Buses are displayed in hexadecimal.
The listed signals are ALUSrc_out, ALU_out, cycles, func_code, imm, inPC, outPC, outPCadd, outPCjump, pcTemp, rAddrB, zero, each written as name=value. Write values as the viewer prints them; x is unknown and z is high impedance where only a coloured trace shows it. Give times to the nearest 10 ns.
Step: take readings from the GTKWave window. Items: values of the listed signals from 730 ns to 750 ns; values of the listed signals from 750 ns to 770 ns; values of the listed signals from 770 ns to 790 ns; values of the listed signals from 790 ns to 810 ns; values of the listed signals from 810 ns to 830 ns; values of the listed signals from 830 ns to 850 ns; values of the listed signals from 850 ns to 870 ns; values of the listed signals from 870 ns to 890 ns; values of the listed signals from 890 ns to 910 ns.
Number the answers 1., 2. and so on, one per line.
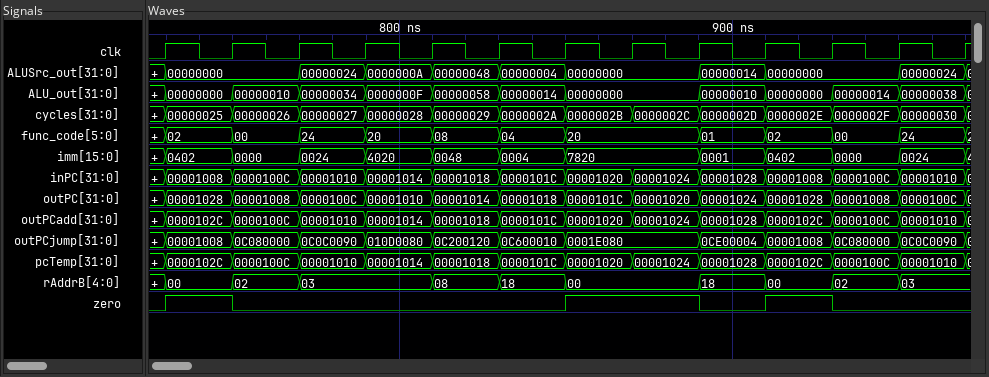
1. ALUSrc_out=00000000, ALU_out=00000000, cycles=00000025, func_code=02, imm=0402, inPC=00001008, outPC=00001028, outPCadd=0000102C, outPCjump=00001008, pcTemp=0000102C, rAddrB=00, zero=1
2. ALUSrc_out=00000000, ALU_out=00000010, cycles=00000026, func_code=00, imm=0000, inPC=0000100C, outPC=00001008, outPCadd=0000100C, outPCjump=0C080000, pcTemp=0000100C, rAddrB=02, zero=0
3. ALUSrc_out=00000024, ALU_out=00000034, cycles=00000027, func_code=24, imm=0024, inPC=00001010, outPC=0000100C, outPCadd=00001010, outPCjump=0C0C0090, pcTemp=00001010, rAddrB=03, zero=0
4. ALUSrc_out=0000000A, ALU_out=0000000F, cycles=00000028, func_code=20, imm=4020, inPC=00001014, outPC=00001010, outPCadd=00001014, outPCjump=010D0080, pcTemp=00001014, rAddrB=03, zero=0
5. ALUSrc_out=00000048, ALU_out=00000058, cycles=00000029, func_code=08, imm=0048, inPC=00001018, outPC=00001014, outPCadd=00001018, outPCjump=0C200120, pcTemp=00001018, rAddrB=08, zero=0
6. ALUSrc_out=00000004, ALU_out=00000014, cycles=0000002A, func_code=04, imm=0004, inPC=0000101C, outPC=00001018, outPCadd=0000101C, outPCjump=0C600010, pcTemp=0000101C, rAddrB=18, zero=0
7. ALUSrc_out=00000000, ALU_out=00000000, cycles=0000002B, func_code=20, imm=7820, inPC=00001020, outPC=0000101C, outPCadd=00001020, outPCjump=0001E080, pcTemp=00001020, rAddrB=00, zero=1
8. ALUSrc_out=00000000, ALU_out=00000000, cycles=0000002C, func_code=20, imm=7820, inPC=00001024, outPC=00001020, outPCadd=00001024, outPCjump=0001E080, pcTemp=00001024, rAddrB=00, zero=1
9. ALUSrc_out=00000014, ALU_out=00000010, cycles=0000002D, func_code=01, imm=0001, inPC=00001028, outPC=00001024, outPCadd=00001028, outPCjump=0CE00004, pcTemp=00001028, rAddrB=18, zero=0
